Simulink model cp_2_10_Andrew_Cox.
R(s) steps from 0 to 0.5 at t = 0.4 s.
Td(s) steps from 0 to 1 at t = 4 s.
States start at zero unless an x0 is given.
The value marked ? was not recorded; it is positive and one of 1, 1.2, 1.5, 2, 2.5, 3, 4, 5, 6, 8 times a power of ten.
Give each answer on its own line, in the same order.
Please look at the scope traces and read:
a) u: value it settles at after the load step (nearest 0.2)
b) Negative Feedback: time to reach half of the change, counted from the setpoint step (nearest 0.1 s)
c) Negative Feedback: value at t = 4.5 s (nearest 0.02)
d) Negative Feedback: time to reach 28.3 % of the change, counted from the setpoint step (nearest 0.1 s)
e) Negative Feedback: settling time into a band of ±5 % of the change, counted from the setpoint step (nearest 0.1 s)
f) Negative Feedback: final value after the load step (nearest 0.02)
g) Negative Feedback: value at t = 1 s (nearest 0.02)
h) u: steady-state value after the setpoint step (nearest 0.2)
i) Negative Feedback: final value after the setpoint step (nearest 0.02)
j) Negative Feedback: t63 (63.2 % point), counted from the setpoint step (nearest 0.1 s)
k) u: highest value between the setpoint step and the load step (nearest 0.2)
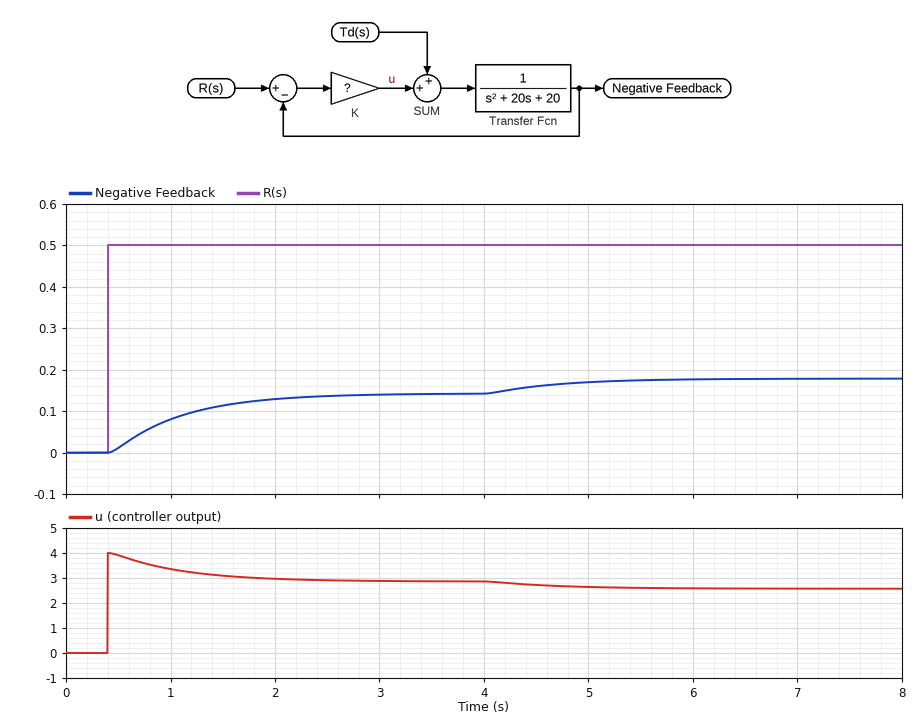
2.6
0.5 s
0.16
0.3 s
2.0 s
0.18
0.08
2.8
0.14
0.7 s
4.0
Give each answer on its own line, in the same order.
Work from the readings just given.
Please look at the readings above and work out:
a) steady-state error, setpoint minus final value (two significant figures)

0.36
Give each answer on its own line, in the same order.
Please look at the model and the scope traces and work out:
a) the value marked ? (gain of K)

8
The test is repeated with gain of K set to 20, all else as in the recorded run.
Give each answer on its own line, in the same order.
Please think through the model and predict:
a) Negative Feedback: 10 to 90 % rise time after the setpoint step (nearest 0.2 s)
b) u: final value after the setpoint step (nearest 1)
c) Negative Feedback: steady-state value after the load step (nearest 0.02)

1.0 s
5
0.28
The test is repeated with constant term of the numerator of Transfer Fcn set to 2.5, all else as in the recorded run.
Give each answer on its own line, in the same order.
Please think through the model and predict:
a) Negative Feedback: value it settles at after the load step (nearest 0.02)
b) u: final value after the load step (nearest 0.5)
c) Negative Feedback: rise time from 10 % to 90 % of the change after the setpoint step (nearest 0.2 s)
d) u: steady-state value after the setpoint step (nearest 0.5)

0.32
1.5
1.0 s
2.0
